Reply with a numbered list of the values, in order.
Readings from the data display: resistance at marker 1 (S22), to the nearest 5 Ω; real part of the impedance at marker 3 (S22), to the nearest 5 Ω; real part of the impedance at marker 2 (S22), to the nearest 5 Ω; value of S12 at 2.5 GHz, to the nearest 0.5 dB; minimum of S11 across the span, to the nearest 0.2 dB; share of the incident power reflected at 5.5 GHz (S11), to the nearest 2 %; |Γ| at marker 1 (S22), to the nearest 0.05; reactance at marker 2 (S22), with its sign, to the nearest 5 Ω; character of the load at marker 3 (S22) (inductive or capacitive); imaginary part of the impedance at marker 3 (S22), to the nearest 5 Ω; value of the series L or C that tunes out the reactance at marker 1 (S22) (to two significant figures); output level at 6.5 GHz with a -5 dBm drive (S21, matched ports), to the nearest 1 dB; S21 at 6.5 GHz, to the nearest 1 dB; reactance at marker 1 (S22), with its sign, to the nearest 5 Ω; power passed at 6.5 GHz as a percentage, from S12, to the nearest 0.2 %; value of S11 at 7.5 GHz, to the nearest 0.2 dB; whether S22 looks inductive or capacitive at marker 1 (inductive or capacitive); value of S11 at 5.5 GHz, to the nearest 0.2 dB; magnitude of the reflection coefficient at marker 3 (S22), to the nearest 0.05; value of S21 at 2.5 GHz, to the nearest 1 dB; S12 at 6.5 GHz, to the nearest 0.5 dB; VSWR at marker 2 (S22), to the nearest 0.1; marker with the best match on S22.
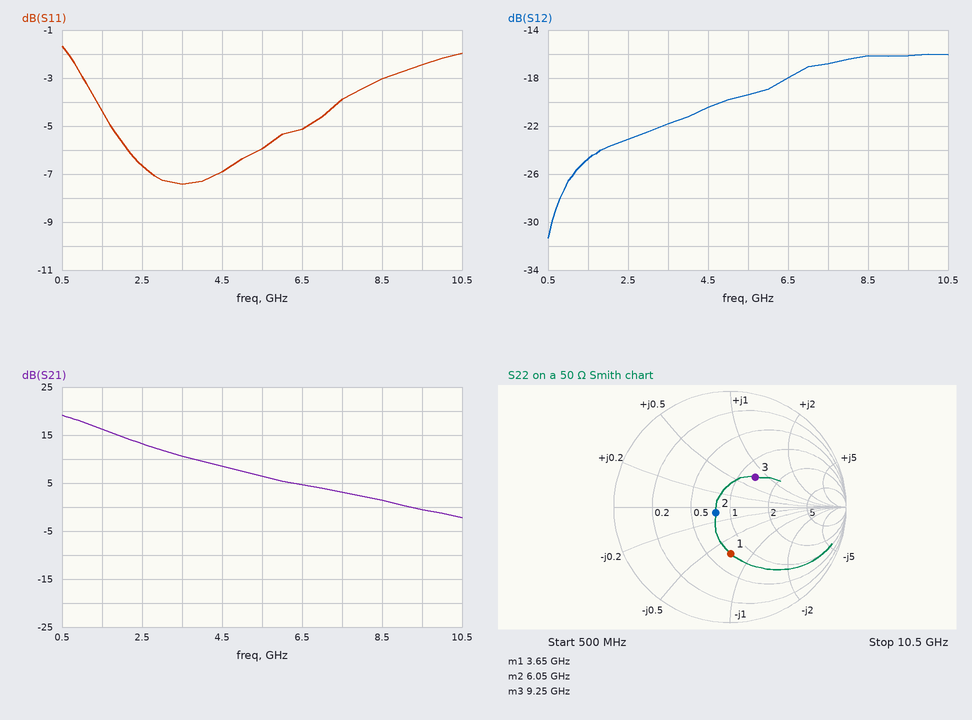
1. 35 Ω
2. 65 Ω
3. 40 Ω
4. -23.0 dB
5. -7.4 dB
6. 26 %
7. 0.40
8. -5 Ω
9. inductive
10. +40 Ω
11. 1.5 nH
12. 0 dBm
13. 5 dB
14. -35 Ω
15. 1.6 %
16. -3.8 dB
17. capacitive
18. -6.0 dB
19. 0.35
20. 13 dB
21. -18.0 dB
22. 1.3
23. marker 2
